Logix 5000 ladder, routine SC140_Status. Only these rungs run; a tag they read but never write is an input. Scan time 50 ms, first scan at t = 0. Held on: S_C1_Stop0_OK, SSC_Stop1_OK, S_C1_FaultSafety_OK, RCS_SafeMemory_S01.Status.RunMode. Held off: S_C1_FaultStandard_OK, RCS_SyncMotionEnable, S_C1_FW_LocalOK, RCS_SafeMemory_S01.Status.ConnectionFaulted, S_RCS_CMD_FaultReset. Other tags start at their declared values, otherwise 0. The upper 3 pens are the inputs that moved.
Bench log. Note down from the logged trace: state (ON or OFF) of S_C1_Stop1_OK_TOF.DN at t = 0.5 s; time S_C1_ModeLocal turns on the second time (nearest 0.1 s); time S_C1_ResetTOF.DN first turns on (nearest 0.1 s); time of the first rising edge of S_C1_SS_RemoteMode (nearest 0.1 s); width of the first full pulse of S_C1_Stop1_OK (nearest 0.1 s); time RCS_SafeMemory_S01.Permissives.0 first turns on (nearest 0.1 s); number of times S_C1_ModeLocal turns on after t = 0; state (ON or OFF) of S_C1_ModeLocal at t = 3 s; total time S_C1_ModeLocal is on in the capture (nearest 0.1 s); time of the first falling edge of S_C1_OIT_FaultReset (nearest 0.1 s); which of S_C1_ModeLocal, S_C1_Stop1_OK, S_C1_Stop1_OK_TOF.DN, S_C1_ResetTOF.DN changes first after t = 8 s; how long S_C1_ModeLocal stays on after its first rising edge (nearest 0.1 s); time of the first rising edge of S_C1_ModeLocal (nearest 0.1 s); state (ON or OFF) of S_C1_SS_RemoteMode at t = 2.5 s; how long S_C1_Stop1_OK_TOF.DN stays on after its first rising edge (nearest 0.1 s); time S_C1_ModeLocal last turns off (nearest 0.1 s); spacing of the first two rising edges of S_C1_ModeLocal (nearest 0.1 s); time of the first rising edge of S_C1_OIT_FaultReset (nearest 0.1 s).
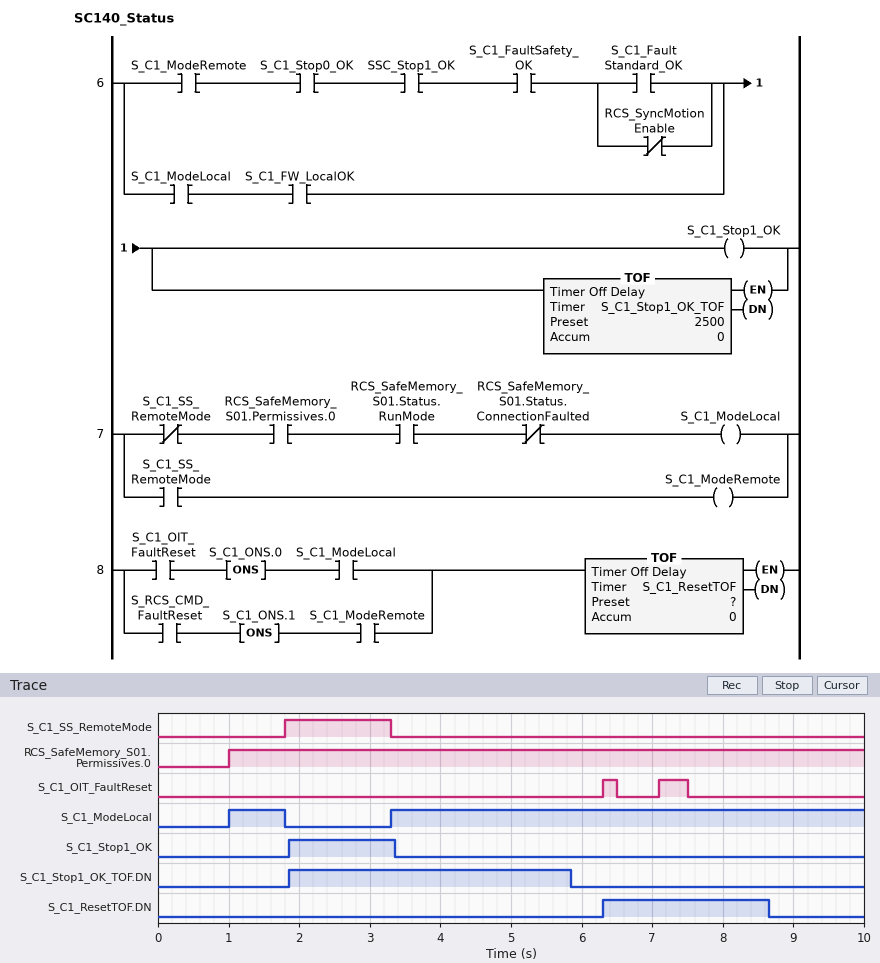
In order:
OFF
3.3 s
6.3 s
1.8 s
1.5 s
1.0 s
2
OFF
7.5 s
6.5 s
S_C1_ResetTOF.DN
0.8 s
1.0 s
ON
4.0 s
1.8 s
2.3 s
6.3 s
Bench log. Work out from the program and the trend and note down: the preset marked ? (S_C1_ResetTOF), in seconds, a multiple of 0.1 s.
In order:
1.5 s
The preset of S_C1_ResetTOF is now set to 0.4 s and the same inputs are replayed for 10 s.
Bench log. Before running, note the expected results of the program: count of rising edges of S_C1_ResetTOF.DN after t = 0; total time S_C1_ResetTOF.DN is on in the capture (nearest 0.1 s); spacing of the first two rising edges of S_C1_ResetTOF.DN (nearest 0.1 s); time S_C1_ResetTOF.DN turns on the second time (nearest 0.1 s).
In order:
2
0.9 s
0.8 s
7.1 s
